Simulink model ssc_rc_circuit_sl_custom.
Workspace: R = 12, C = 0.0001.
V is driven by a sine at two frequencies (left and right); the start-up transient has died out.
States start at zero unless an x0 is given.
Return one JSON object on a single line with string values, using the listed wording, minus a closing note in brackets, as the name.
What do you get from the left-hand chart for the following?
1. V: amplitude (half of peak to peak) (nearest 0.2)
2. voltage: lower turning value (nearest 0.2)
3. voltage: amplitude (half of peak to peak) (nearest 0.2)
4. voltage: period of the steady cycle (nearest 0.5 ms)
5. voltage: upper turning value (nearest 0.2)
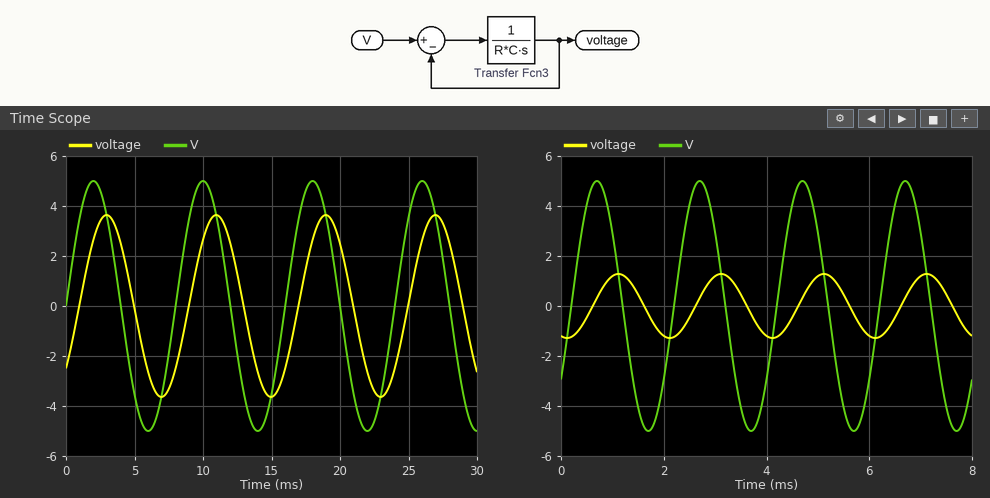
{"V: amplitude (half of peak to peak)": "5.0", "voltage: lower turning value": "-3.6", "voltage: amplitude (half of peak to peak)": "3.6", "voltage: period of the steady cycle": "8.0 ms", "voltage: upper turning value": "3.6"}
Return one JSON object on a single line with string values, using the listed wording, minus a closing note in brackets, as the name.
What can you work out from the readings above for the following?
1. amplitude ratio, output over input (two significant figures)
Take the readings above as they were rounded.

{"amplitude ratio, output over input": "0.72"}
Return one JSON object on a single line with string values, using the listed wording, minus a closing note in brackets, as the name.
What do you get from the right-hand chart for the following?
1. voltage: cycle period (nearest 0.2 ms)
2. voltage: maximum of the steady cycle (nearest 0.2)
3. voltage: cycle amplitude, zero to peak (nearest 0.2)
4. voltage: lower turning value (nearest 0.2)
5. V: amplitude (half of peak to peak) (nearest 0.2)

{"voltage: cycle period": "2.0 ms", "voltage: maximum of the steady cycle": "1.2", "voltage: cycle amplitude, zero to peak": "1.2", "voltage: lower turning value": "-1.2", "V: amplitude (half of peak to peak)": "5.0"}
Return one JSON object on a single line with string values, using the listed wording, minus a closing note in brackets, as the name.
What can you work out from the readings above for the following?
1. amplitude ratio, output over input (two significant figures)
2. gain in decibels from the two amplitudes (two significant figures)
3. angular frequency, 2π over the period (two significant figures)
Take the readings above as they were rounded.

{"amplitude ratio, output over input": "0.24", "gain in decibels from the two amplitudes": "-12 dB", "angular frequency, 2π over the period": "3.1 rad/ms"}
